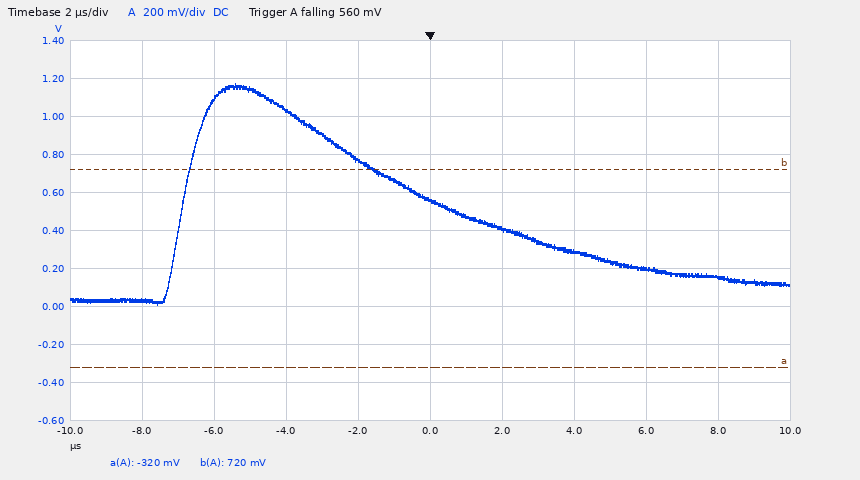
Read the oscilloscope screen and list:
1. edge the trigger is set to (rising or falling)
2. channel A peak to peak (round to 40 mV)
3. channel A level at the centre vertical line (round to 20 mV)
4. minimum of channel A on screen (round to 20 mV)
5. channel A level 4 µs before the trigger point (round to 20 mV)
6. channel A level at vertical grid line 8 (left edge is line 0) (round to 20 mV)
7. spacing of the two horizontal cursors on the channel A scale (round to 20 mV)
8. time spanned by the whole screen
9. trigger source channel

falling
1.16 V
560 mV
20 mV
1.04 V
200 mV
1.04 V
20 µs
channel A
